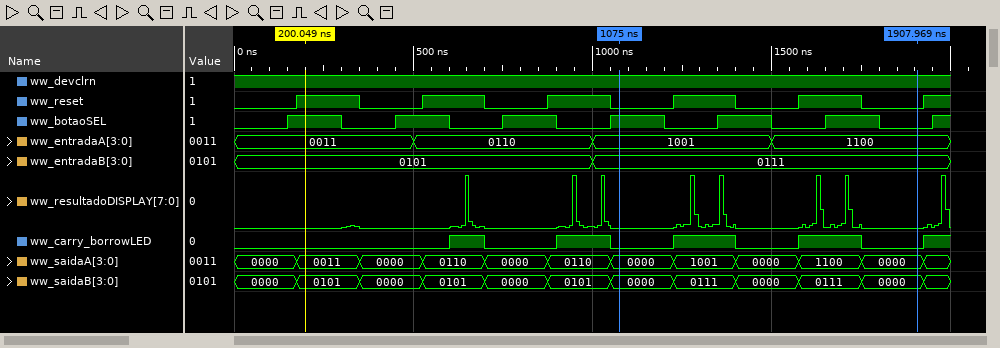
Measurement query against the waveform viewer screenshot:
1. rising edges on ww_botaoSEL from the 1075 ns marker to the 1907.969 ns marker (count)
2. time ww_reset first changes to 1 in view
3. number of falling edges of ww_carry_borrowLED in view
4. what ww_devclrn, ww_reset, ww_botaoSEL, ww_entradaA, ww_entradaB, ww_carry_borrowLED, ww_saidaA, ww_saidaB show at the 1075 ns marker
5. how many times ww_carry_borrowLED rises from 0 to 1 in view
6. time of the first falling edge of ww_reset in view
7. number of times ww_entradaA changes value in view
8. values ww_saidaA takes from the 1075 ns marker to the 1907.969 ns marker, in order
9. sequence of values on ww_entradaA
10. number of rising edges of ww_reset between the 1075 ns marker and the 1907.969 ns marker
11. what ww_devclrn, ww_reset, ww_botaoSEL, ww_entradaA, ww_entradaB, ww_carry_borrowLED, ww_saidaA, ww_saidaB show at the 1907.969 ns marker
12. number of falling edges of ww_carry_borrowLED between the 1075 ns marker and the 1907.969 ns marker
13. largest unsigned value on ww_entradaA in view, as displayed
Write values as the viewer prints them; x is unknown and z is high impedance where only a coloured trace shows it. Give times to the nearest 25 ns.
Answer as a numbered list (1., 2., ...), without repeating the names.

1. 2
2. 175 ns
3. 4
4. ww_devclrn=1, ww_reset=0, ww_botaoSEL=1, ww_entradaA=1001, ww_entradaB=0111, ww_carry_borrowLED=0, ww_saidaA=0000, ww_saidaB=0000
5. 5
6. 350 ns
7. 3
8. 0000, 1001, 0000, 1100, 0000
9. 0011, 0110, 1001, 1100
10. 2
11. ww_devclrn=1, ww_reset=0, ww_botaoSEL=0, ww_entradaA=1100, ww_entradaB=0111, ww_carry_borrowLED=0, ww_saidaA=0000, ww_saidaB=0000
12. 2
13. 1100
